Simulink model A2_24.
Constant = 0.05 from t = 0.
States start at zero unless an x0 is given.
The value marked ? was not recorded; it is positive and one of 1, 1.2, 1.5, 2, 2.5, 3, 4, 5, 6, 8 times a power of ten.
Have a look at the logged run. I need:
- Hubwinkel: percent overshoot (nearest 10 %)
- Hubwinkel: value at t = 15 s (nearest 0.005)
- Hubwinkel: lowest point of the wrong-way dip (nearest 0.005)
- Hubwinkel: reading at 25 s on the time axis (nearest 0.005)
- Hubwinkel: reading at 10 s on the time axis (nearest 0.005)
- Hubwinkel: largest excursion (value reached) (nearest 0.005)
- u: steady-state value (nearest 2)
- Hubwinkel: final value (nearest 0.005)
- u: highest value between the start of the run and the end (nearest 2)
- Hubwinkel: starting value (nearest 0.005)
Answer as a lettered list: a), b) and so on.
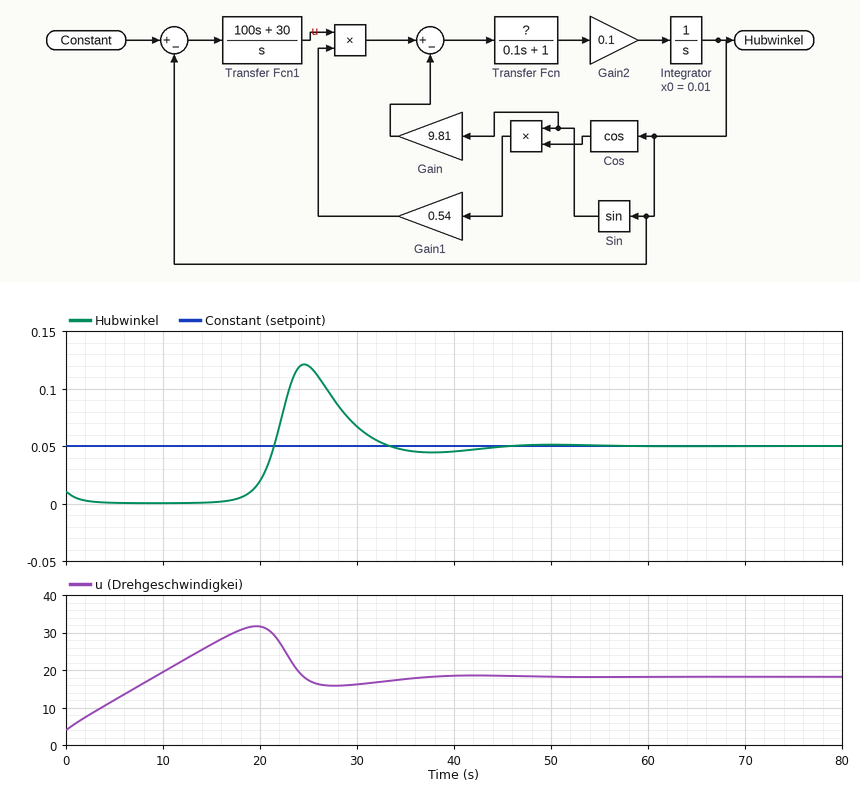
a) 180 %
b) 0.000
c) 0.000
d) 0.120
e) 0.000
f) 0.120
g) 18
h) 0.050
i) 32
j) 0.010
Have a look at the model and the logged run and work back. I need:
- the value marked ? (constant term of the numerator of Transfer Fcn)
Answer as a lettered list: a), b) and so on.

a) 1
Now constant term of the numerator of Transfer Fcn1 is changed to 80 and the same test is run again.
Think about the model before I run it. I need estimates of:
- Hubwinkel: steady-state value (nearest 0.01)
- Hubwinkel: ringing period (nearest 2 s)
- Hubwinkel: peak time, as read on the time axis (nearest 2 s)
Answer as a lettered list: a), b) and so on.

a) 0.05
b) 14 s
c) 12 s
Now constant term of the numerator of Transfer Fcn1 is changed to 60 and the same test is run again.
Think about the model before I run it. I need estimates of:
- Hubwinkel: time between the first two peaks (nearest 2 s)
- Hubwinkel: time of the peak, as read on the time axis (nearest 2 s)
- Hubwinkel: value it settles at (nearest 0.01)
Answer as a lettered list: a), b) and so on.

a) 16 s
b) 14 s
c) 0.05
